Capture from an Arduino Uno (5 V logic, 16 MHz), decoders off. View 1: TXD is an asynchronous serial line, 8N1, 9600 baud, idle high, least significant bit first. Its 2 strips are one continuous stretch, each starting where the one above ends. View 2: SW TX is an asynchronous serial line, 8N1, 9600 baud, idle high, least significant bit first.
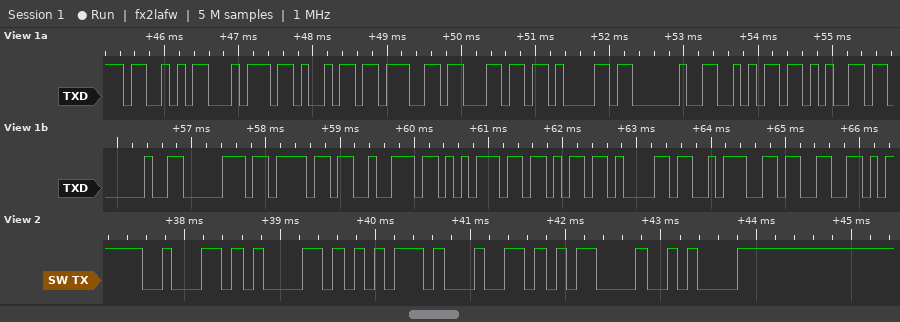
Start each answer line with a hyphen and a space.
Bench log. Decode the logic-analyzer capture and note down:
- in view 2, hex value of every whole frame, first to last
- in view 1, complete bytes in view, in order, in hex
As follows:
- 62 61 75 64 0D 0A
- 53 74 69 67 6C 61 20 6A 65 20 70 6F 72 75 6B 61 3A 33
